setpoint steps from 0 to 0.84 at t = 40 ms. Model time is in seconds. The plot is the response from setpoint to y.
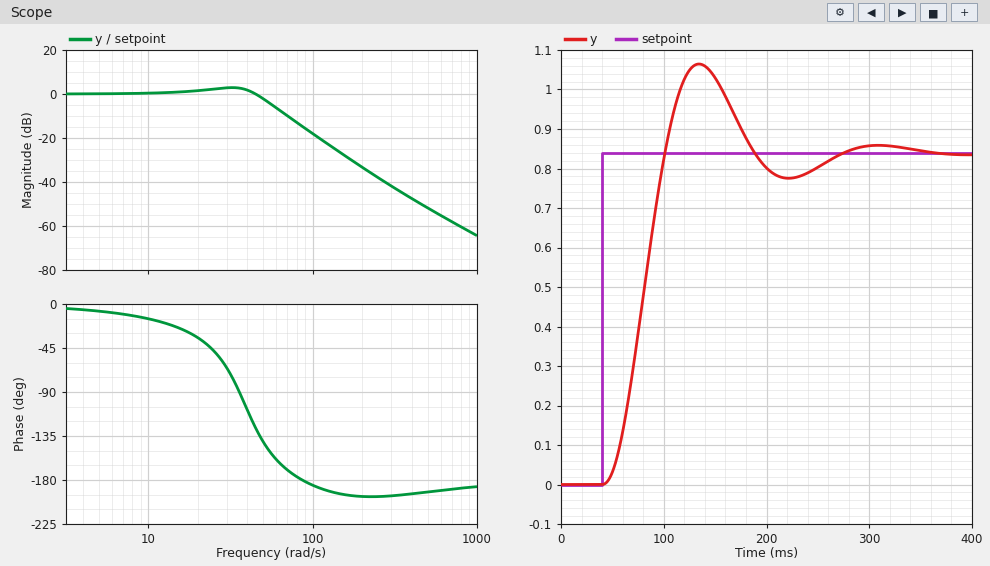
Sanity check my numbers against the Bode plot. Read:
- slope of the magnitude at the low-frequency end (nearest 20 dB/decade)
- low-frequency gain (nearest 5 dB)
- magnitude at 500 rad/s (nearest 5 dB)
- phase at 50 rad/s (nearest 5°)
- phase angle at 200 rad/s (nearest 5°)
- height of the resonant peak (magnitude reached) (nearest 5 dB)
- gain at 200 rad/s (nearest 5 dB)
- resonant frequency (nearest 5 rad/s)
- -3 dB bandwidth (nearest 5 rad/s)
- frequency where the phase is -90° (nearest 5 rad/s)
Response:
0 dB/decade
0 dB
-50 dB
-140°
-195°
5 dB
-35 dB
30 rad/s
50 rad/s
35 rad/s
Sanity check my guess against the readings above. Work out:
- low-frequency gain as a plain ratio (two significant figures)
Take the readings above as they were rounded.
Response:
1.0
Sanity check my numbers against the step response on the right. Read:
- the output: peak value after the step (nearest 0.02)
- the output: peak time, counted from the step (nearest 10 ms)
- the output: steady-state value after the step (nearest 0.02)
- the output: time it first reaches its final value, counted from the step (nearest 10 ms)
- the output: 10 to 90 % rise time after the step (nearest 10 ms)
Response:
1.06
90 ms
0.84
60 ms
40 ms
